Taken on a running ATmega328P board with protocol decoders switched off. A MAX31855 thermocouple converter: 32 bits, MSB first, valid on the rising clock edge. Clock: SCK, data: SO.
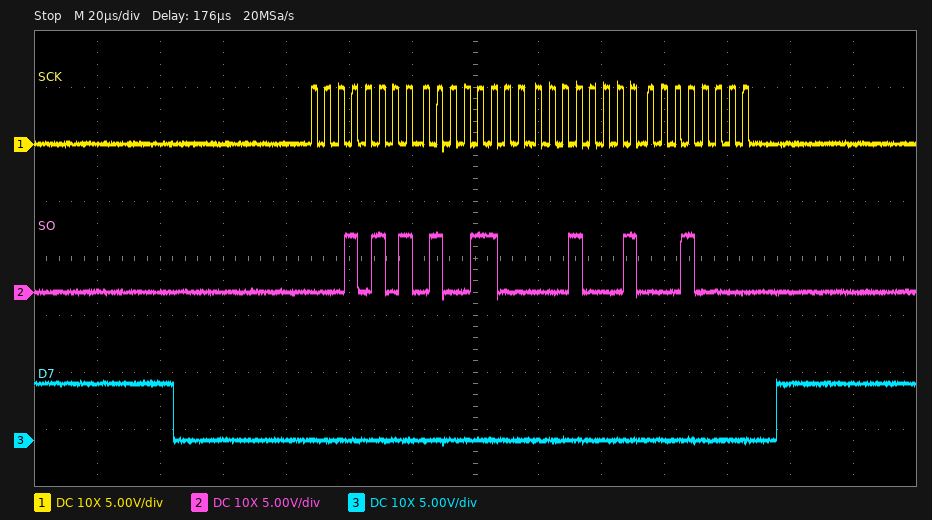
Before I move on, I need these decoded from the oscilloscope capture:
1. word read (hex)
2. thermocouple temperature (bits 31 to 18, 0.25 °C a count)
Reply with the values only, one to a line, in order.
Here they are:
0x154C1110
340.75 °C
